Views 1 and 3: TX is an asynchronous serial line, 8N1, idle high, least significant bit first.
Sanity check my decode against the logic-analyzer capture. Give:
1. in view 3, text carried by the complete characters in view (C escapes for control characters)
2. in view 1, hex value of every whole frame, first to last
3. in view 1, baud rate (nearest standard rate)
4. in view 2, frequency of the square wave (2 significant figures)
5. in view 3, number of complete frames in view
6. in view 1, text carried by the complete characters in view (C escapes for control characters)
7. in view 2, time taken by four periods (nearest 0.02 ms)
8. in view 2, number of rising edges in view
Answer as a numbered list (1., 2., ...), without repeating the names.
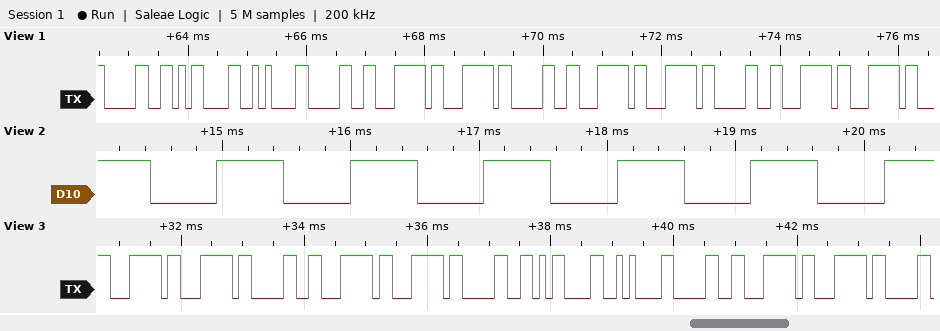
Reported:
1. "||0||0\r\n0||"
2. 30 0D 0A 30 7C 7C 30 7C 7C 30 7C 7C
3. 9600 baud
4. 960 Hz
5. 11
6. "0\r\n0||0||0||"
7. 4.16 ms
8. 6
